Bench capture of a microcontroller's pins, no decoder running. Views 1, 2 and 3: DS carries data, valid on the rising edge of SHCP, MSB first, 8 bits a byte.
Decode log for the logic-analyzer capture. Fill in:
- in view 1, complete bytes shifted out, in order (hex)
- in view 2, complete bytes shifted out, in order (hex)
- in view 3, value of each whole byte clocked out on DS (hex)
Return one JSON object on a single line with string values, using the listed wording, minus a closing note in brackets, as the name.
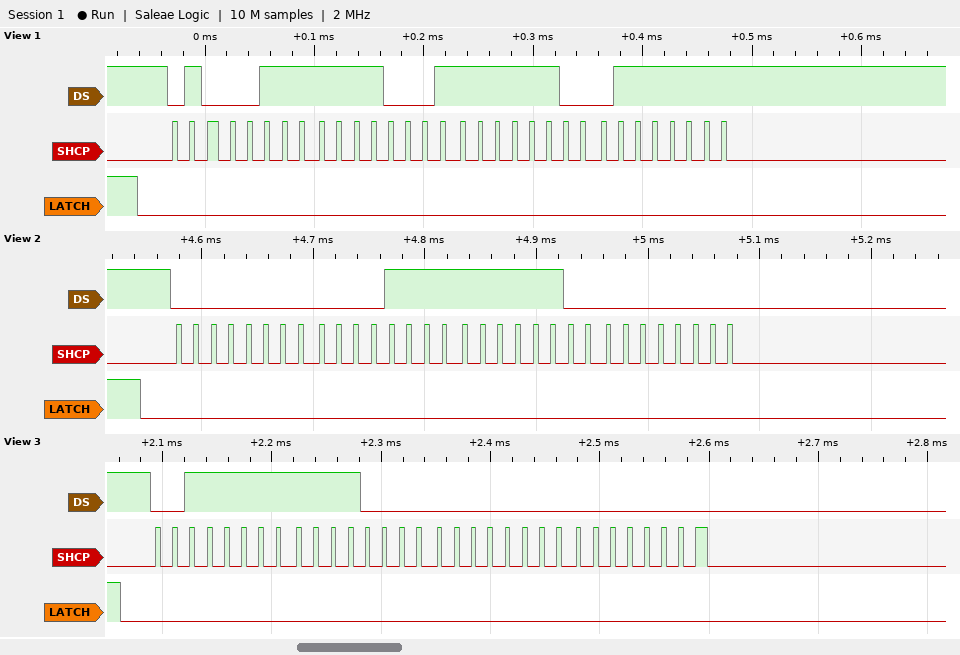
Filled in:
{"in view 1, complete bytes shifted out, in order": "47 F1 FC 7F", "in view 2, complete bytes shifted out, in order": "00 0F FC 00", "in view 3, value of each whole byte clocked out on DS": "0x3F 0xF0 0x00 0x00"}
